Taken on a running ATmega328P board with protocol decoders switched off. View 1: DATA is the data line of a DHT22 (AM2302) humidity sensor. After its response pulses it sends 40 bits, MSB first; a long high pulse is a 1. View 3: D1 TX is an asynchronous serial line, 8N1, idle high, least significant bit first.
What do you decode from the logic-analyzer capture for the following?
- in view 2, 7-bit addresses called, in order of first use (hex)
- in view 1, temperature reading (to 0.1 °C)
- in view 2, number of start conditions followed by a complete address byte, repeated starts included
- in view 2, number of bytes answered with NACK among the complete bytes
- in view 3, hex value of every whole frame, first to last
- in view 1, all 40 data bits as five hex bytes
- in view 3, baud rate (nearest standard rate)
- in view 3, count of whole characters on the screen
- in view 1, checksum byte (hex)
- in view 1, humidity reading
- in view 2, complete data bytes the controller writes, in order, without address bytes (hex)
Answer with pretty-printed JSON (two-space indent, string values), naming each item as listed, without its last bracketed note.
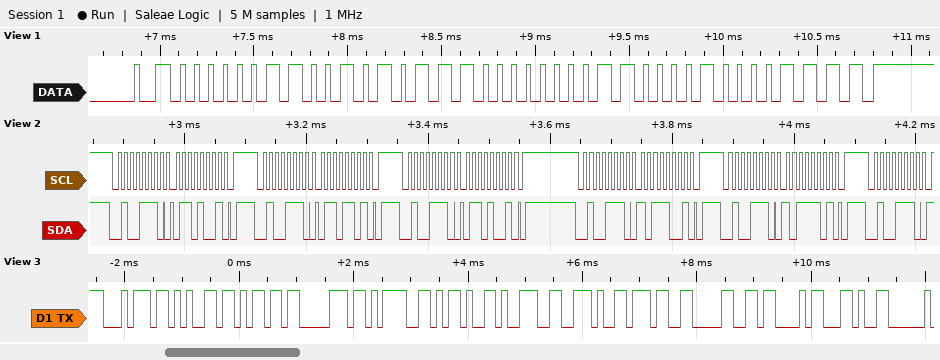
{
  "in view 2, 7-bit addresses called, in order of first use": "0x27",
  "in view 1, temperature reading": "-9.7 °C",
  "in view 2, number of start conditions followed by a complete address byte, repeated starts included": "6",
  "in view 2, number of bytes answered with NACK among the complete bytes": "0",
  "in view 3, hex value of every whole frame, first to last": "74 65 6D 70 3D 2D 39 2E 37 30 43 2C",
  "in view 1, all 40 data bits as five hex bytes": "03 2B 80 61 0F",
  "in view 3, baud rate": "9600 baud",
  "in view 3, count of whole characters on the screen": "12",
  "in view 1, checksum byte": "0x0F",
  "in view 1, humidity reading": "81.1 %",
  "in view 2, complete data bytes the controller writes, in order, without address bytes": "69 6D 69 B9 BD"
}
